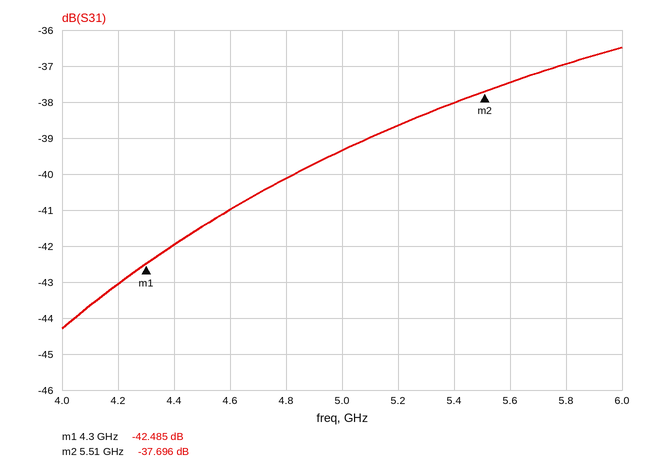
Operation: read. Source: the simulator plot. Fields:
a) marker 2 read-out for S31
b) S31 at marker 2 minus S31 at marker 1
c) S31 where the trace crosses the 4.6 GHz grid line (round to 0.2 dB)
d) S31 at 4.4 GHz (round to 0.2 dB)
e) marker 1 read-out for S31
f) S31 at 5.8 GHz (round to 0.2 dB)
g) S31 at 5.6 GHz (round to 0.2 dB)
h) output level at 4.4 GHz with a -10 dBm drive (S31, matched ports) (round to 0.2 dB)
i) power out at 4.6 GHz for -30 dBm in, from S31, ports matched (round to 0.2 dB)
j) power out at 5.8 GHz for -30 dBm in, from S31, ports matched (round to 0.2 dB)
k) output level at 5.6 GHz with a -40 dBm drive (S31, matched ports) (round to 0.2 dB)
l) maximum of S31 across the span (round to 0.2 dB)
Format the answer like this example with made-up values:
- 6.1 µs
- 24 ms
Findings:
- -37.696 dB
- 4.789 dB
- -41.0 dB
- -42.0 dB
- -42.485 dB
- -37.0 dB
- -37.4 dB
- -52.0 dBm
- -71.0 dBm
- -67.0 dBm
- -77.4 dBm
- -36.4 dB
